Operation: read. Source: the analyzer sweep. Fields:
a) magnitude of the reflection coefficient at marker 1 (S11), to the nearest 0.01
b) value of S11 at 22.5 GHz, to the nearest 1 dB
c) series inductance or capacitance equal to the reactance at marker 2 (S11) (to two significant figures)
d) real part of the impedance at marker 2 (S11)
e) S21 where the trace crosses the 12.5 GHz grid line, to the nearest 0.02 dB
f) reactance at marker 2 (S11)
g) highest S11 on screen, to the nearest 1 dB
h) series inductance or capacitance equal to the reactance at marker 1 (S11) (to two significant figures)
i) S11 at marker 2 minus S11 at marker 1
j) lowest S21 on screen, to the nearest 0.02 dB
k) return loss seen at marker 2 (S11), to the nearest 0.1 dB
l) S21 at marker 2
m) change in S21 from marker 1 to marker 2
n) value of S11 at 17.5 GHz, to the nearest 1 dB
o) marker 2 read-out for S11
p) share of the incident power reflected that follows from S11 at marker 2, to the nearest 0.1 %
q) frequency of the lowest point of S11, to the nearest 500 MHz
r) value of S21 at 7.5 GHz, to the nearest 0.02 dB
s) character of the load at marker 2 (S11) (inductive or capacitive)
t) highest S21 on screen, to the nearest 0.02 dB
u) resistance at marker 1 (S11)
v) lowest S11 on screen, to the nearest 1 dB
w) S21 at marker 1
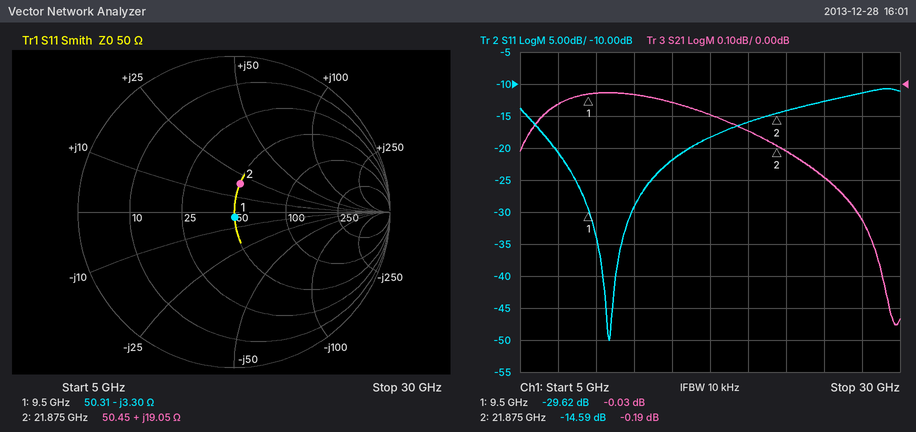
0.03
-14 dB
140 pH
50.45 Ω
-0.04 dB
+19.05 Ω
-11 dB
5.1 pF
15.03 dB
-0.76 dB
14.6 dB
-0.19 dB
-0.16 dB
-18 dB
-14.59 dB
3.5 %
11.0 GHz
-0.06 dB
inductive
-0.02 dB
50.31 Ω
-50 dB
-0.03 dB
